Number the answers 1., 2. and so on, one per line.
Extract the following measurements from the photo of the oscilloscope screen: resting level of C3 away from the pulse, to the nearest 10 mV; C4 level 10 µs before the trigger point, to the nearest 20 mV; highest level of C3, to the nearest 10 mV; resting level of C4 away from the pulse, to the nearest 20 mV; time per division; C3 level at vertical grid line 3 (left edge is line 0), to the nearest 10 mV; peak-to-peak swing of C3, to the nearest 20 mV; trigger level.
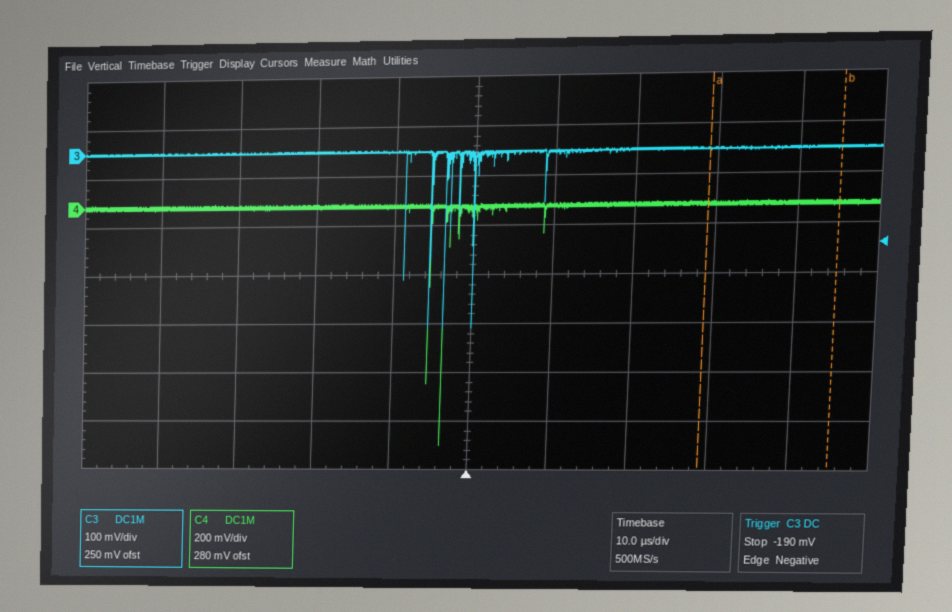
1. 0 mV
2. 0 mV
3. 0 mV
4. 0 mV
5. 10 µs
6. 0 mV
7. 360 mV
8. -190 mV
